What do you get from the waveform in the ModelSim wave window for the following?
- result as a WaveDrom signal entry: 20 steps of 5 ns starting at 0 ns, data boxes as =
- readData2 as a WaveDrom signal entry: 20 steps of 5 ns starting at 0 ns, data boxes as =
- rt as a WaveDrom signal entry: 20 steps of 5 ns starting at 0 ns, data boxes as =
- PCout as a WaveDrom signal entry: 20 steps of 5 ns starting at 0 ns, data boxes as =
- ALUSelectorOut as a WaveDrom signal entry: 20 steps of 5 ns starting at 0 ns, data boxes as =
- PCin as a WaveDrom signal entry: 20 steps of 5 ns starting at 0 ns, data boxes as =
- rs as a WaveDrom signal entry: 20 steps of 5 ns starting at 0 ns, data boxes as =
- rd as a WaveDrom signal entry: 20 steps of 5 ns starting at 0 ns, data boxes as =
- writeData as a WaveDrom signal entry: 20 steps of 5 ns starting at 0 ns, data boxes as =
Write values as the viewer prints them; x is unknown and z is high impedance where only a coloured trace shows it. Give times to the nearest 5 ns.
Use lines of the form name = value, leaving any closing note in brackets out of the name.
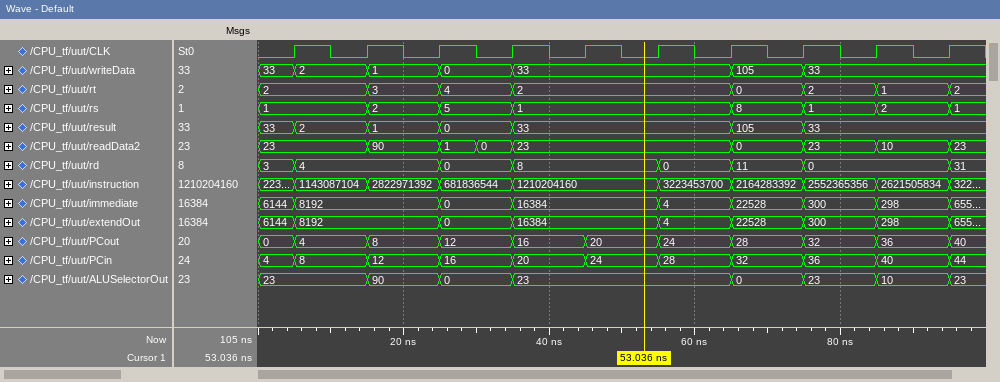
result as a WaveDrom signal entry: 20 steps of 5 ns starting at 0 ns, data boxes as = = {name: 'result', wave: '==.=.=.=.....=.=....', data: '33 2 1 0 33 105 33'}
readData2 as a WaveDrom signal entry: 20 steps of 5 ns starting at 0 ns, data boxes as = = {name: 'readData2', wave: '=..=.===.....=.=.=.=', data: '23 90 1 0 23 0 23 10 23'}
rt as a WaveDrom signal entry: 20 steps of 5 ns starting at 0 ns, data boxes as = = {name: 'rt', wave: '=..=.=.=.....=.=.=.=', data: '2 3 4 2 0 2 1 2'}
PCout as a WaveDrom signal entry: 20 steps of 5 ns starting at 0 ns, data boxes as = = {name: 'PCout', wave: '==.=.=.=.=.=.=.=.=.=', data: '0 4 8 12 16 20 24 28 32 36 40'}
ALUSelectorOut as a WaveDrom signal entry: 20 steps of 5 ns starting at 0 ns, data boxes as = = {name: 'ALUSelectorOut', wave: '=..=.=.=.....=.=.=.=', data: '23 90 0 23 0 23 10 23'}
PCin as a WaveDrom signal entry: 20 steps of 5 ns starting at 0 ns, data boxes as = = {name: 'PCin', wave: '==.=.=.=.=.=.=.=.=.=', data: '4 8 12 16 20 24 28 32 36 40 44'}
rs as a WaveDrom signal entry: 20 steps of 5 ns starting at 0 ns, data boxes as = = {name: 'rs', wave: '=..=.=.=.....=.=.=.=', data: '1 2 5 1 8 1 2 1'}
rd as a WaveDrom signal entry: 20 steps of 5 ns starting at 0 ns, data boxes as = = {name: 'rd', wave: '==...=.=...=.=.=...=', data: '3 4 0 8 0 11 0 31'}
writeData as a WaveDrom signal entry: 20 steps of 5 ns starting at 0 ns, data boxes as = = {name: 'writeData', wave: '==.=.=.=.....=.=....', data: '33 2 1 0 33 105 33'}
